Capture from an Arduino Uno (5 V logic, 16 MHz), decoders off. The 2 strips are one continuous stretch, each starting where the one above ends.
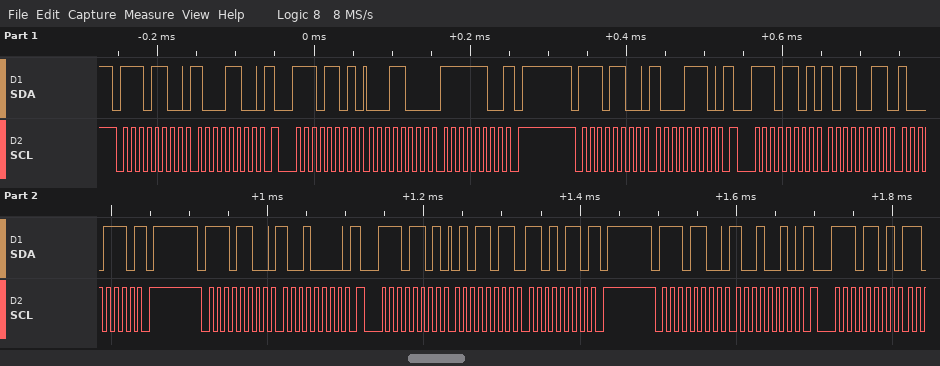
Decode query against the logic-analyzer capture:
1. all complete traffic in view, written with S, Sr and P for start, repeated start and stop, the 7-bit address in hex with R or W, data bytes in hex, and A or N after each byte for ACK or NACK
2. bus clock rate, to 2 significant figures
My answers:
S 76W A 8C A Sr 76R A 18 A FC N P S 76W A 8E A Sr 76R A B3 A 8E N P S 76W A 90 A Sr 76R A 5B A D6 N P S 76W A 92 A Sr 76R A
100 kHz
